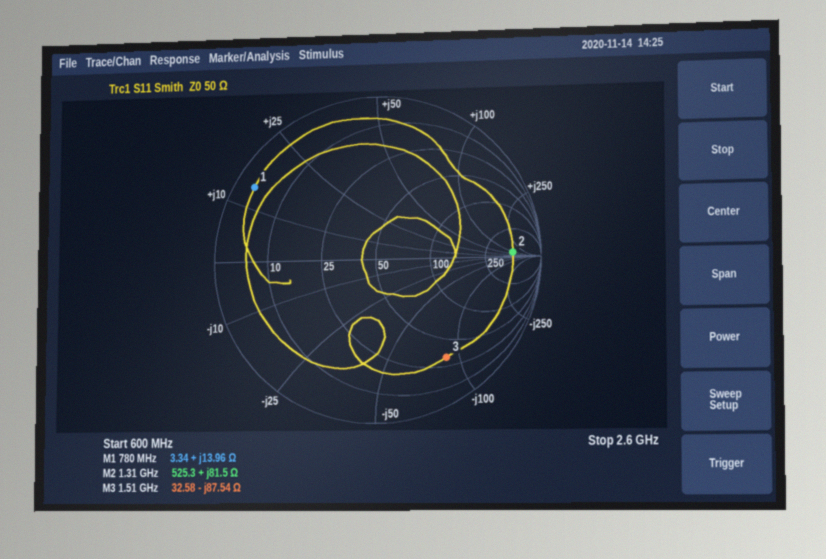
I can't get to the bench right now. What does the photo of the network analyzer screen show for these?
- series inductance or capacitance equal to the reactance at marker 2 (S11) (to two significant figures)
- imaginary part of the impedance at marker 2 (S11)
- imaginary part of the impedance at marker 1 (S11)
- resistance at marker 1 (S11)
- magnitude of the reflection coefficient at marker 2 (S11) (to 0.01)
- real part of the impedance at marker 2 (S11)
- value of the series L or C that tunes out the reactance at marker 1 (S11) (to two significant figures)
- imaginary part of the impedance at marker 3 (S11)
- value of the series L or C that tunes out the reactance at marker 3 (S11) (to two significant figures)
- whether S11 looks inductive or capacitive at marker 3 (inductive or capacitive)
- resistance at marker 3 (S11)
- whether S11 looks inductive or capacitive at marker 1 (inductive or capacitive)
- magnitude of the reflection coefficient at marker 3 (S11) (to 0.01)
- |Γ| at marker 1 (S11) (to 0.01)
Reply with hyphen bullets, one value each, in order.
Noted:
- 9.9 nH
- +81.5 Ω
- +13.96 Ω
- 3.34 Ω
- 0.83
- 525.3 Ω
- 15 pF
- -87.54 Ω
- 9.2 nH
- capacitive
- 32.58 Ω
- inductive
- 0.74
- 0.88
